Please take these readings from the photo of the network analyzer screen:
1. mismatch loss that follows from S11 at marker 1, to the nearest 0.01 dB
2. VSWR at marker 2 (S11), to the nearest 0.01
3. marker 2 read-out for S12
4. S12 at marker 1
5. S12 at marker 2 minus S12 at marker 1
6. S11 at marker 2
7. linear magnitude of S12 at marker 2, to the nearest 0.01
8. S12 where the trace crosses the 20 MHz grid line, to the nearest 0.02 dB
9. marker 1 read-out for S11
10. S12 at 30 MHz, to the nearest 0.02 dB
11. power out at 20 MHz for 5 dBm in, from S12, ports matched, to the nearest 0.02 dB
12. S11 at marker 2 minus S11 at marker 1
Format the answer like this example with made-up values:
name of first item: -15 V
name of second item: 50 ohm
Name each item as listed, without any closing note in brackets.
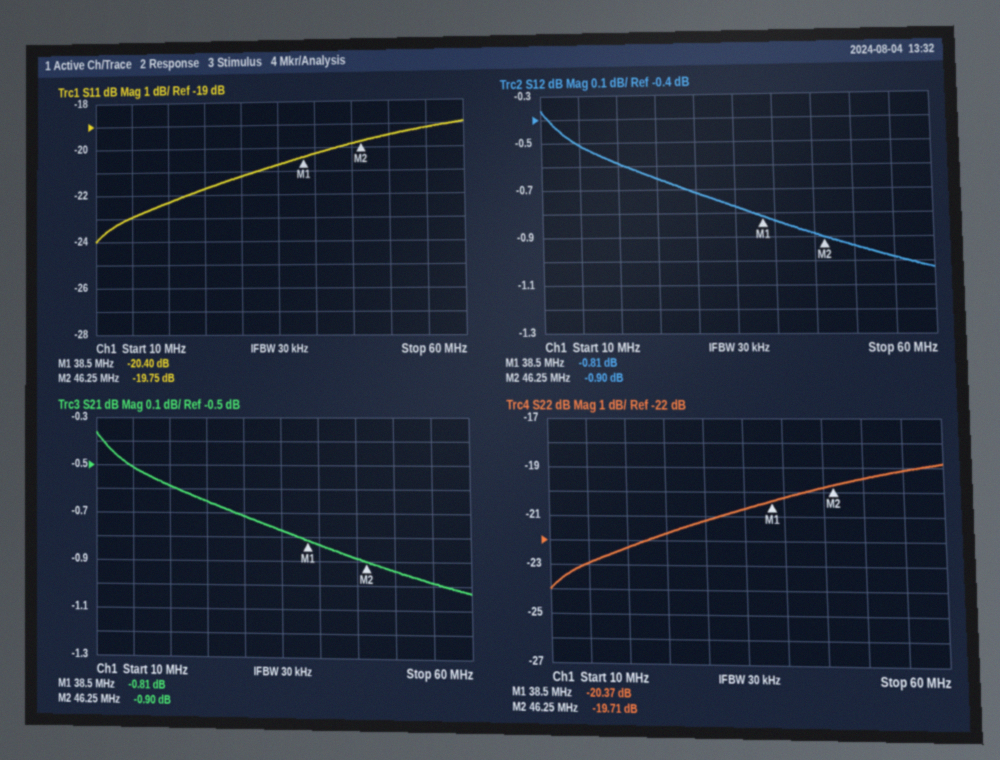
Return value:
mismatch loss that follows from S11 at marker 1, to the nearest 0.01 dB: 0.04 dB
VSWR at marker 2 (S11), to the nearest 0.01: 1.23
marker 2 read-out for S12: -0.90 dB
S12 at marker 1: -0.81 dB
S12 at marker 2 minus S12 at marker 1: -0.09 dB
S11 at marker 2: -19.75 dB
linear magnitude of S12 at marker 2, to the nearest 0.01: 0.90
S12 where the trace crosses the 20 MHz grid line, to the nearest 0.02 dB: -0.58 dB
marker 1 read-out for S11: -20.40 dB
S12 at 30 MHz, to the nearest 0.02 dB: -0.72 dB
power out at 20 MHz for 5 dBm in, from S12, ports matched, to the nearest 0.02 dB: 4.42 dBm
S11 at marker 2 minus S11 at marker 1: 0.65 dB
